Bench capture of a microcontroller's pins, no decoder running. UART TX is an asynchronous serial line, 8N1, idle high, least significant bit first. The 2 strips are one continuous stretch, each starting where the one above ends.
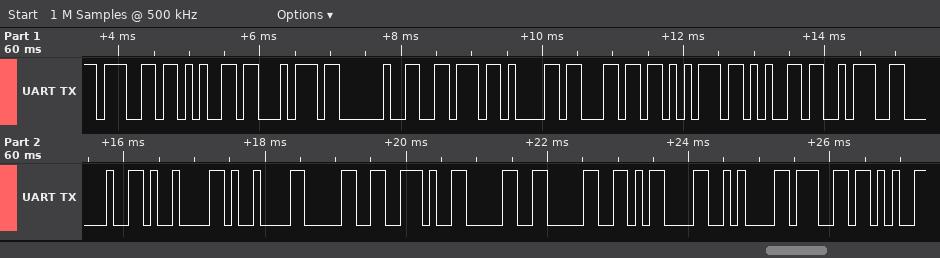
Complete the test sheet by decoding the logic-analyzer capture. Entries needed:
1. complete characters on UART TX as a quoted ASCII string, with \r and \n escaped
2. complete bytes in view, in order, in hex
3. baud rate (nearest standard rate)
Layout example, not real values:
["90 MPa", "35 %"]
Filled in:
["\"get value: \\t\\t0.00\\r\\ng\"", "67 65 74 20 76 61 6C 75 65 3A 20 09 09 30 2E 30 30 0D 0A 67", "9600 baud"]
